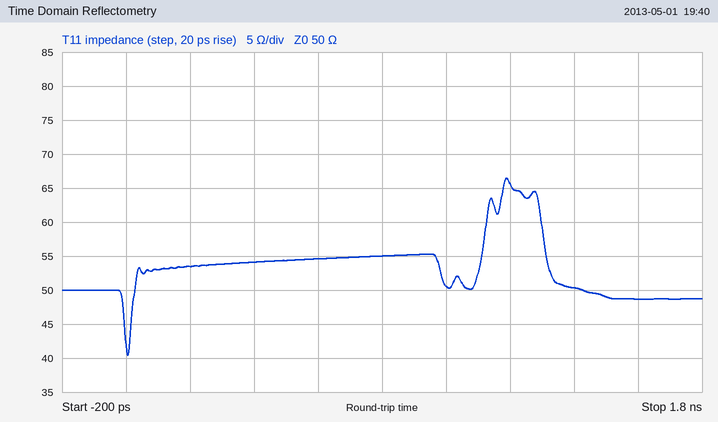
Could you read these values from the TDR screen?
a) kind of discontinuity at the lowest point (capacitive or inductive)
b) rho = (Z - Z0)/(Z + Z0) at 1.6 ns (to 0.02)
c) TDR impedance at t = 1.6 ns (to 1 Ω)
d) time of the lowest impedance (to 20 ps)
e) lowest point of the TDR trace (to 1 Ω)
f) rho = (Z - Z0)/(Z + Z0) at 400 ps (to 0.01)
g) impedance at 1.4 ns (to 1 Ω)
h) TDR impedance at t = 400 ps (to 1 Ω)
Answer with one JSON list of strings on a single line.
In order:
["capacitive", "-0.02", "49 Ω", "0 ps", "40 Ω", "+0.04", "50 Ω", "54 Ω"]
